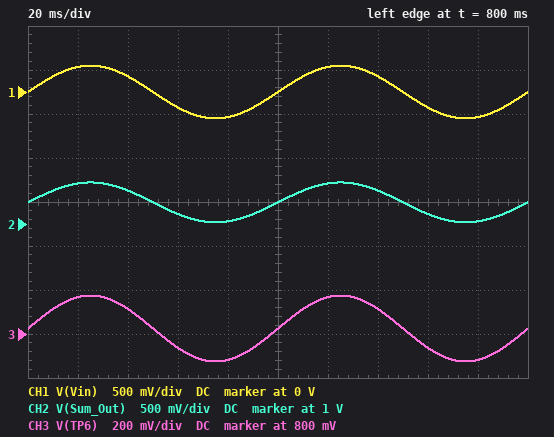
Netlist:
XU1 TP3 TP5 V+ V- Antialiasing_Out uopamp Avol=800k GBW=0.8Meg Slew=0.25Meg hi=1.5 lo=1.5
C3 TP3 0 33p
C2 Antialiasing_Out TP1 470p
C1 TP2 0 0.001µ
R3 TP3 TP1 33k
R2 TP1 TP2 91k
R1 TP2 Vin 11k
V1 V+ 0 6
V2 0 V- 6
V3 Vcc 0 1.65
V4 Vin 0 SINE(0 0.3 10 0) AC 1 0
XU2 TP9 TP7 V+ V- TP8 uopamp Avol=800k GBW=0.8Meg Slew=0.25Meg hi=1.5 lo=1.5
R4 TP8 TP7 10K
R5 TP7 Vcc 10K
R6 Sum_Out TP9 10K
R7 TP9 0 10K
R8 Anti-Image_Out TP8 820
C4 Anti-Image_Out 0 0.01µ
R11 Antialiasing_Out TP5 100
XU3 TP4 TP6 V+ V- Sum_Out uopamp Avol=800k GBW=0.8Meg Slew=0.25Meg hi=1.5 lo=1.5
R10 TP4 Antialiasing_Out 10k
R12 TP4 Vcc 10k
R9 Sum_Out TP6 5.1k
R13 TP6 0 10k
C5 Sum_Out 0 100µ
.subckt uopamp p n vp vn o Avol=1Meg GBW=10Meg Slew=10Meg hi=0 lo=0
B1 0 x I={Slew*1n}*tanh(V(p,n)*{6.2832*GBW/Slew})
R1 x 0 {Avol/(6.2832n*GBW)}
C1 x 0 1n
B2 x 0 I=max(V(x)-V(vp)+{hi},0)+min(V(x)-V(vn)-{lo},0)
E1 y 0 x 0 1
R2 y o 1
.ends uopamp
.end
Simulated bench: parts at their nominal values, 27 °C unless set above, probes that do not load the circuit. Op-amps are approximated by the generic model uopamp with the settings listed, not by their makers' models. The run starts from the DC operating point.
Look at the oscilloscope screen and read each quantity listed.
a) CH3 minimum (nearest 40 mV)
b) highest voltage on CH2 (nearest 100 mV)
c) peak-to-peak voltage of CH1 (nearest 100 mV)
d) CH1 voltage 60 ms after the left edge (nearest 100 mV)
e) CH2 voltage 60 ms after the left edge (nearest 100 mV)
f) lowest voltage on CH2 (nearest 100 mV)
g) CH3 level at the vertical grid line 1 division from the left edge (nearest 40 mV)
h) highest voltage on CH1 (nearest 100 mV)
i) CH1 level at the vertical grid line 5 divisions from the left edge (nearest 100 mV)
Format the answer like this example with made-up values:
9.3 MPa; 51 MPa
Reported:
680 mV; 1.5 V; 600 mV; -200 mV; 1.1 V; 1.0 V; 960 mV; 300 mV; 0 V
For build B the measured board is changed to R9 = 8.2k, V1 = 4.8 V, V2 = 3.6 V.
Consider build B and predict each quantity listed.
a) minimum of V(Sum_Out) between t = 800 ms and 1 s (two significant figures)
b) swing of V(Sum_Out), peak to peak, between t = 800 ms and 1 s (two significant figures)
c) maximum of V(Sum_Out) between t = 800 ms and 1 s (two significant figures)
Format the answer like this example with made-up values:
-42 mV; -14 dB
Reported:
1.2 V; 550 mV; 1.8 V
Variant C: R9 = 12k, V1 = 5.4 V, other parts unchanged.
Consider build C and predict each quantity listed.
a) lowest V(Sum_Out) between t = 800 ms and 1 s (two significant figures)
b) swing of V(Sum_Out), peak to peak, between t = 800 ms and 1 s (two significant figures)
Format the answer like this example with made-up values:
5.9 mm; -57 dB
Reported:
1.5 V; 660 mV
